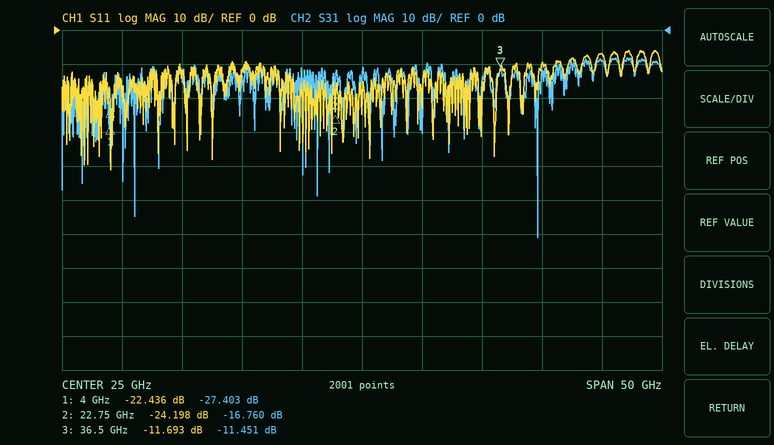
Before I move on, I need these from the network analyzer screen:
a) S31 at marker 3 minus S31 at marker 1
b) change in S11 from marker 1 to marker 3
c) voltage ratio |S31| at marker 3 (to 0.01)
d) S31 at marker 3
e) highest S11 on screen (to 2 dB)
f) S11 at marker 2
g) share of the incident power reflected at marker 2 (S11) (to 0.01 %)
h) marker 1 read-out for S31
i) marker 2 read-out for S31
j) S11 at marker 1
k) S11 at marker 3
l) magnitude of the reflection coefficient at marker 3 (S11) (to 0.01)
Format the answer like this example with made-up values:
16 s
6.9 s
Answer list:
15.952 dB
10.743 dB
0.27
-11.451 dB
-6 dB
-24.198 dB
0.38 %
-27.403 dB
-16.760 dB
-22.436 dB
-11.693 dB
0.26
